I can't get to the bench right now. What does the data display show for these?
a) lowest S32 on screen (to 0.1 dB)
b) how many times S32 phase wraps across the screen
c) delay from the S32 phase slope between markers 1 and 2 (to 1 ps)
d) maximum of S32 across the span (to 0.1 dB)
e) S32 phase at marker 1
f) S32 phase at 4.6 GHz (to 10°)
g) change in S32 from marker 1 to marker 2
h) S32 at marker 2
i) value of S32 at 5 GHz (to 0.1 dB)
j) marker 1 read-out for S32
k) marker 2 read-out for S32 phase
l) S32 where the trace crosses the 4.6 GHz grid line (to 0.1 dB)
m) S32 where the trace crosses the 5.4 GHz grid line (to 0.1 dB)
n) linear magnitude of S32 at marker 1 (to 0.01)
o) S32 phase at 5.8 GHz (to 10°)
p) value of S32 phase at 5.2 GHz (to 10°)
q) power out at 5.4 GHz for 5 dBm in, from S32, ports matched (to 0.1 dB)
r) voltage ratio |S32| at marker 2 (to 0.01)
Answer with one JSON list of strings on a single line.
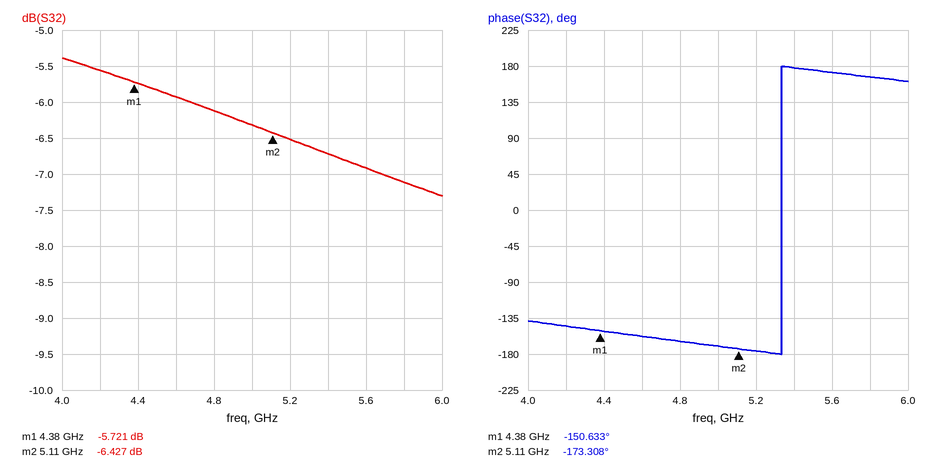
["-7.3 dB", "1", "86 ps", "-5.4 dB", "-150.633°", "-160°", "-0.706 dB", "-6.427 dB", "-6.3 dB", "-5.721 dB", "-173.308°", "-5.9 dB", "-6.7 dB", "0.52", "170°", "-180°", "-1.7 dBm", "0.48"]
